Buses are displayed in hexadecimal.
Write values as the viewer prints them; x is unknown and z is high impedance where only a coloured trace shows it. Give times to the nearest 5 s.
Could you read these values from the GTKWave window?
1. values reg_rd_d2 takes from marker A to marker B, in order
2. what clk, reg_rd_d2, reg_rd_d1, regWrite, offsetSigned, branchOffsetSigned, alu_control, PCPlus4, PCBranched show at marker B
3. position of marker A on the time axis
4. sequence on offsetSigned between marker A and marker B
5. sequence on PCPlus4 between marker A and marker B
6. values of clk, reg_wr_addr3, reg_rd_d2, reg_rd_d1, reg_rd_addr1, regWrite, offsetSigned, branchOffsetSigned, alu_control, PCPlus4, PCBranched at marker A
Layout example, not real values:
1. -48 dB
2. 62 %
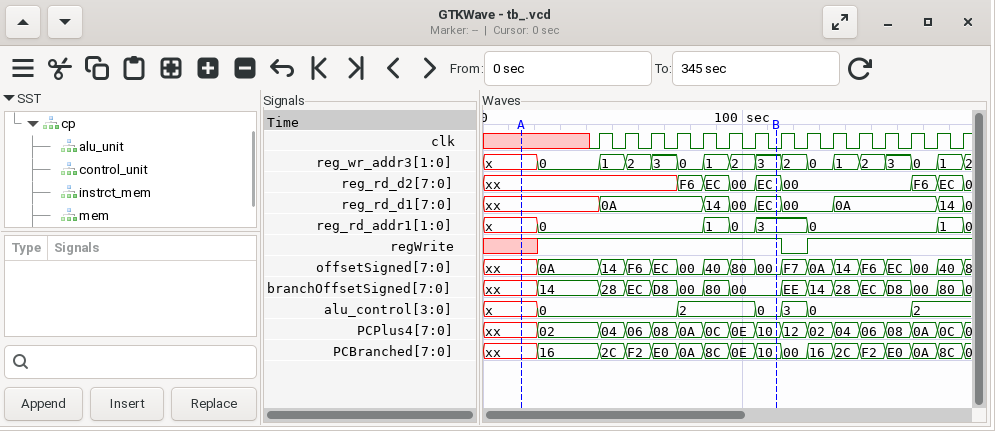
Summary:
1. xx, F6, EC, 00, EC
2. clk=0, reg_rd_d2=EC, reg_rd_d1=EC, regWrite=1, offsetSigned=00, branchOffsetSigned=00, alu_control=0, PCPlus4=10, PCBranched=10
3. 15 s
4. xx, 0A, 14, F6, EC, 00, 40, 80, 00
5. xx, 02, 04, 06, 08, 0A, 0C, 0E, 10
6. clk=x, reg_wr_addr3=x, reg_rd_d2=xx, reg_rd_d1=xx, reg_rd_addr1=x, regWrite=x, offsetSigned=xx, branchOffsetSigned=xx, alu_control=x, PCPlus4=xx, PCBranched=xx
